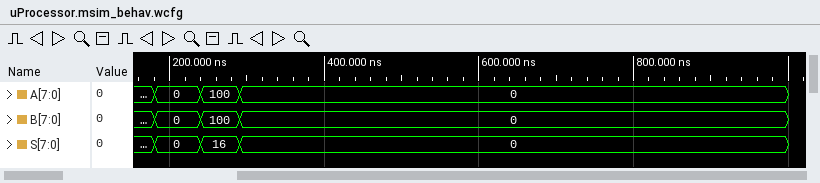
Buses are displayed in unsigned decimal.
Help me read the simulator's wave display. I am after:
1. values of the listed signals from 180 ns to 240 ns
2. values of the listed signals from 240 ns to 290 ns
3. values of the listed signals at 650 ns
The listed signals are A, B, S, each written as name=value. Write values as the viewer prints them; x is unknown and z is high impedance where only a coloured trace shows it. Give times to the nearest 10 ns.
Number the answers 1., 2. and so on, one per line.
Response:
1. A=0, B=0, S=0
2. A=100, B=100, S=16
3. A=0, B=0, S=0
